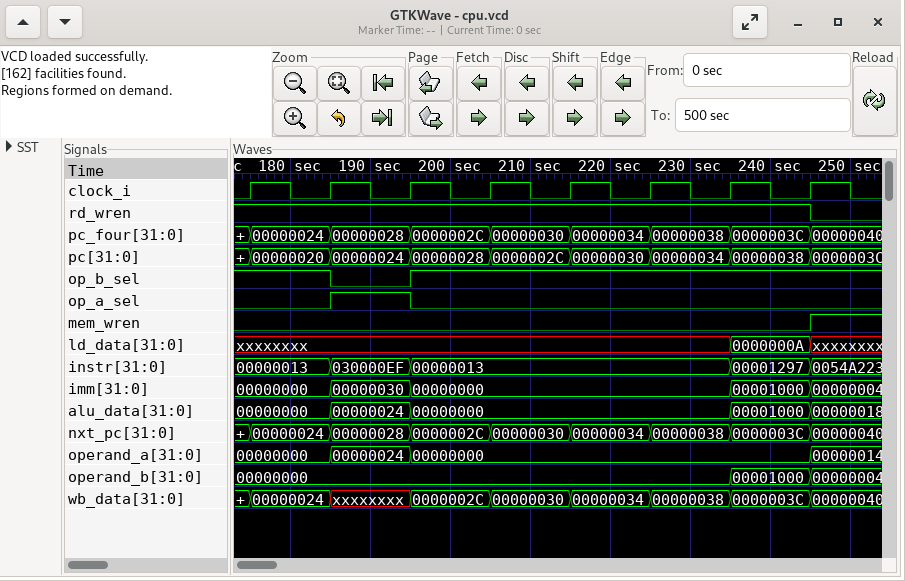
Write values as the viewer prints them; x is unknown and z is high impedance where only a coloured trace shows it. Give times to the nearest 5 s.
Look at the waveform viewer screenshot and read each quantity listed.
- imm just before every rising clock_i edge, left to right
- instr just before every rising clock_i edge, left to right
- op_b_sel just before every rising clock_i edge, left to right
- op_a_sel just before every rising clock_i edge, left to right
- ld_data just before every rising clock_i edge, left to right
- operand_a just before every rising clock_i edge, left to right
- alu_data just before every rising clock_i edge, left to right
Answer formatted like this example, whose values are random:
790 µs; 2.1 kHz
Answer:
00000000, 00000000, 00000030, 00000000, 00000000, 00000000, 00000000, 00001000; 00000013, 00000013, 030000EF, 00000013, 00000013, 00000013, 00000013, 00001297; 1 1 0 1 1 1 1 1; 0 0 1 0 0 0 0 0; xxxxxxxx, xxxxxxxx, xxxxxxxx, xxxxxxxx, xxxxxxxx, xxxxxxxx, xxxxxxxx, 0000000A; 00000000, 00000000, 00000024, 00000000, 00000000, 00000000, 00000000, 00000000; 00000000, 00000000, 00000024, 00000000, 00000000, 00000000, 00000000, 00001000
